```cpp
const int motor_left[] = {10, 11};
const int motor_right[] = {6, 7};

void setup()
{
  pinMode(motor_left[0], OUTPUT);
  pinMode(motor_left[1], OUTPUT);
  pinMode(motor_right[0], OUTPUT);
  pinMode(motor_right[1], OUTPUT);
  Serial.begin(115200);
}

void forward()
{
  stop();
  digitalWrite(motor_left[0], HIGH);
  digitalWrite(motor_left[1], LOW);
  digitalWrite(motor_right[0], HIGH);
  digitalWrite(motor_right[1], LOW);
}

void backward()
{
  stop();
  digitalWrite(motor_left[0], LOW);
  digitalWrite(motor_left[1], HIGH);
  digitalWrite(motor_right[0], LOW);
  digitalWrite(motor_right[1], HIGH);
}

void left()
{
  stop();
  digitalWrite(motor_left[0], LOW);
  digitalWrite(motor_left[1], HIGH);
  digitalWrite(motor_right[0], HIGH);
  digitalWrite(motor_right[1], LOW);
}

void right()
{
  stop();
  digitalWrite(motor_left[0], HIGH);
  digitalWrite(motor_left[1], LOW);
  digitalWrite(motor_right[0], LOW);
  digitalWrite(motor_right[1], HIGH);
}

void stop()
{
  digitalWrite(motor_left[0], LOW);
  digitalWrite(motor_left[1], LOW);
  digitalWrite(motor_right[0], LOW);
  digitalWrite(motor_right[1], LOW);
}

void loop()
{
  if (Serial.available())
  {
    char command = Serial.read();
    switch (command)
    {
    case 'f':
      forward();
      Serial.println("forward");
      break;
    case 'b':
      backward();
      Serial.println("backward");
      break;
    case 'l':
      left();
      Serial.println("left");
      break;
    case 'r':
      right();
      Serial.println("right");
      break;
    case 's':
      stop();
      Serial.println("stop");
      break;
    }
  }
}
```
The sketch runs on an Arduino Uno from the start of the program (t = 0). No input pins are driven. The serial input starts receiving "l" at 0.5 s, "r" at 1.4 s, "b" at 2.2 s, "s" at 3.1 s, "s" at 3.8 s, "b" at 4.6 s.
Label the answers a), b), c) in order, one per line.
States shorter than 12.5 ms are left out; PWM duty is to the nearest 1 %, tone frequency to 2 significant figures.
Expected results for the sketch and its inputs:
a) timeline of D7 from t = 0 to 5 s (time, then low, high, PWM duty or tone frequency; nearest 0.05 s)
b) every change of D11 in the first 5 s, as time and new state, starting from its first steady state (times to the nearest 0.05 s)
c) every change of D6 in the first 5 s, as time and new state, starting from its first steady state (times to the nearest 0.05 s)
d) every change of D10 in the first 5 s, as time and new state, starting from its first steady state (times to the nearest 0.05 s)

a) 0 s low; 1.4 s high; 3.1 s low; 4.6 s high
b) 0 s low; 0.5 s high; 1.4 s low; 2.2 s high; 3.1 s low; 4.6 s high
c) 0 s low; 0.5 s high; 1.4 s low
d) 0 s low; 1.4 s high; 2.2 s low
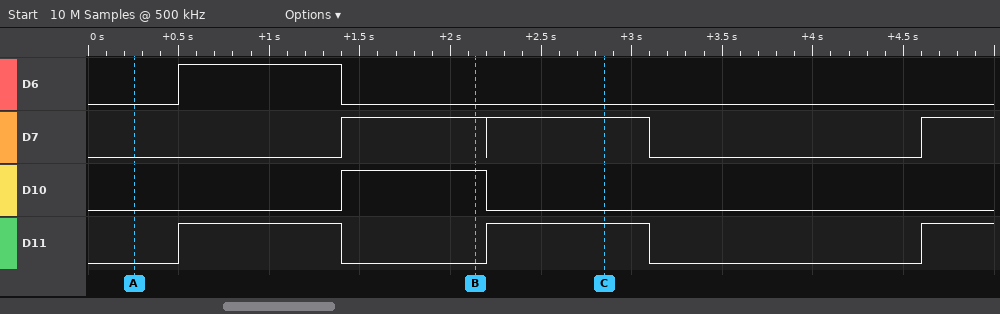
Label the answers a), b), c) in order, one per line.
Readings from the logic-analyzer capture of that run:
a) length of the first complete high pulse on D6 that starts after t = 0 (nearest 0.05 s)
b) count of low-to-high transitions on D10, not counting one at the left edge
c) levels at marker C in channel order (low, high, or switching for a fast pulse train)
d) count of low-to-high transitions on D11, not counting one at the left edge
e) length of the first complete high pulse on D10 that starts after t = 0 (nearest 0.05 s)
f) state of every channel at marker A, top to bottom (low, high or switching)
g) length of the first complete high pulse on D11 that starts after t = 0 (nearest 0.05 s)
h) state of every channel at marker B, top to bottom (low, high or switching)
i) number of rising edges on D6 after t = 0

a) 0.90 s
b) 1
c) D6 low, D7 high, D10 low, D11 high
d) 3
e) 0.80 s
f) D6 low, D7 low, D10 low, D11 low
g) 0.90 s
h) D6 low, D7 high, D10 high, D11 low
i) 1
